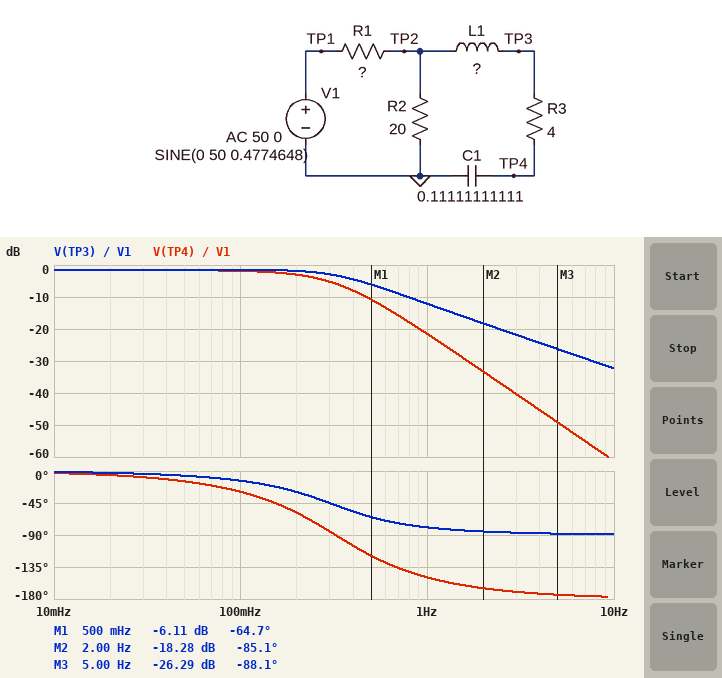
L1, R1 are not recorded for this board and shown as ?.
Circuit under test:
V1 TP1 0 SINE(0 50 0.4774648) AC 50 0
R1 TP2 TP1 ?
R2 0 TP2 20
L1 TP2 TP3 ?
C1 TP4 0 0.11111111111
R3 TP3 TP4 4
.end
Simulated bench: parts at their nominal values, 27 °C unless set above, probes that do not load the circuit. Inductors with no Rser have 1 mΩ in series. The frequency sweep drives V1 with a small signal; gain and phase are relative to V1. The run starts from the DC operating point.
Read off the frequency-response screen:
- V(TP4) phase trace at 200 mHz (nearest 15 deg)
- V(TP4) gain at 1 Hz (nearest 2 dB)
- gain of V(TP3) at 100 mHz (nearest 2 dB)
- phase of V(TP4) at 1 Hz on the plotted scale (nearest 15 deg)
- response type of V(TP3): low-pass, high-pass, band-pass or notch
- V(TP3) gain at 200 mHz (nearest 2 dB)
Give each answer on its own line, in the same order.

-60 deg
-22 dB
-2 dB
-150 deg
low-pass
-2 dB
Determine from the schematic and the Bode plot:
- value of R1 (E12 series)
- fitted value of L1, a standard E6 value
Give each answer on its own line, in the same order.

3.9 Ω
2.2 H
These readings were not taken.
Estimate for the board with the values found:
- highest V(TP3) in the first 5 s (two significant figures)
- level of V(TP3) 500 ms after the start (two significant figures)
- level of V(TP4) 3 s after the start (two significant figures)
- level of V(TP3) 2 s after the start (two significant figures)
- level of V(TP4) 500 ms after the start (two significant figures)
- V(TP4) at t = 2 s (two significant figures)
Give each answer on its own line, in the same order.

29 V
19 V
9.6 V
-26 V
6.2 V
-11 V
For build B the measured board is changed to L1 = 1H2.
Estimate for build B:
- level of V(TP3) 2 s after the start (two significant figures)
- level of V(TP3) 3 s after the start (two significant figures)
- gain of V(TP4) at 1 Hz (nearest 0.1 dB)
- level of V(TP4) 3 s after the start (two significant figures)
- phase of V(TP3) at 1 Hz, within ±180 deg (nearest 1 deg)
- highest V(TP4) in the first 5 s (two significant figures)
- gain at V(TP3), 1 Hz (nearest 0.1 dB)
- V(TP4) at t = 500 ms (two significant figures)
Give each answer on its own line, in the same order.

-24 V
26 V
-18.0 dB
15 V
-60 deg
22 V
-8.5 dB
8.6 V
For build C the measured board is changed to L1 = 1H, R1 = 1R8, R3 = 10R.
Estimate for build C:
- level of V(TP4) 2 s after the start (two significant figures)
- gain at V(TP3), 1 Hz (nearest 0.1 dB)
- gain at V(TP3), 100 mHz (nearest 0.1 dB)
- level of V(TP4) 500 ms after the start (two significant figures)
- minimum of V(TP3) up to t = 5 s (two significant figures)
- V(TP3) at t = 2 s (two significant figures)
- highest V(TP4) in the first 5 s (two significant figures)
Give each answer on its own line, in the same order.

-8.9 V
-2.7 dB
-1.0 dB
7.6 V
-41 V
-22 V
17 V
